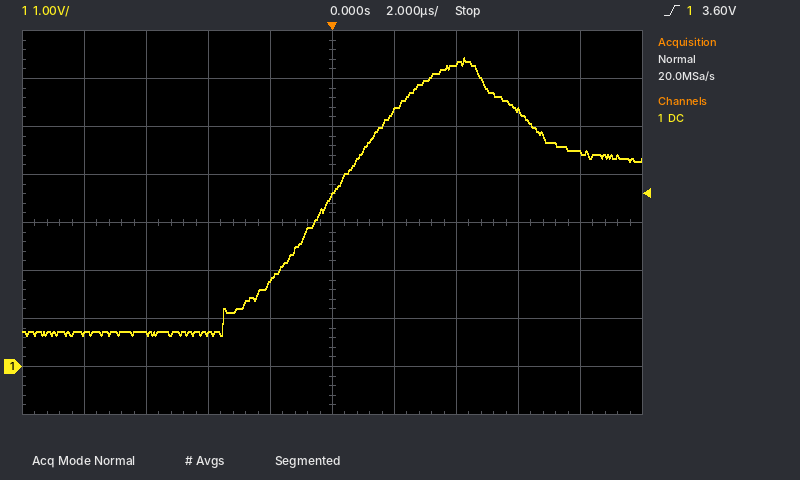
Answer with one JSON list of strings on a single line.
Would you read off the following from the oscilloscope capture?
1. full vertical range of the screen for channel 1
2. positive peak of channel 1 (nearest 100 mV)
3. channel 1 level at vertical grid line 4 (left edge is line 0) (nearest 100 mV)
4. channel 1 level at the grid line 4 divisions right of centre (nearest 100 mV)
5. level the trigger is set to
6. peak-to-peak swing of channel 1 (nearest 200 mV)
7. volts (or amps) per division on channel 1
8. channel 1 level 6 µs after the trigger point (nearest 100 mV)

["8 V", "6.4 V", "1.8 V", "4.5 V", "3.60 V", "5.8 V", "1 V", "5.3 V"]
